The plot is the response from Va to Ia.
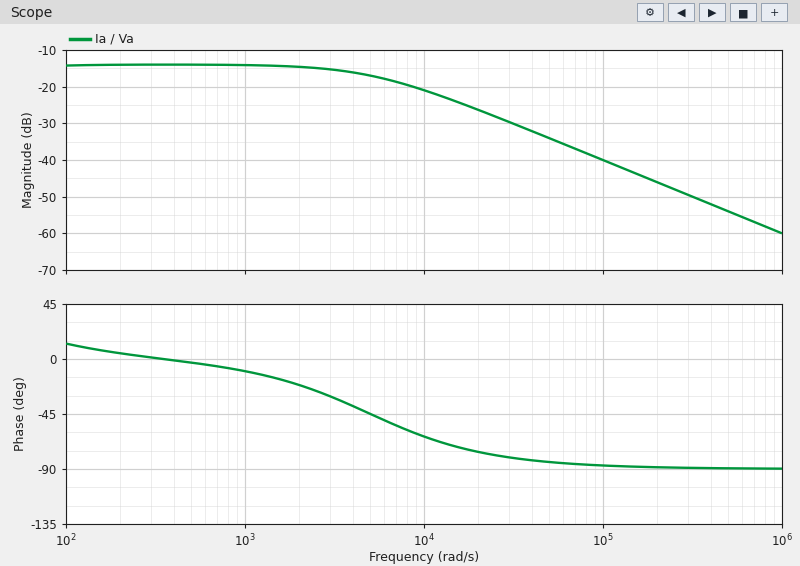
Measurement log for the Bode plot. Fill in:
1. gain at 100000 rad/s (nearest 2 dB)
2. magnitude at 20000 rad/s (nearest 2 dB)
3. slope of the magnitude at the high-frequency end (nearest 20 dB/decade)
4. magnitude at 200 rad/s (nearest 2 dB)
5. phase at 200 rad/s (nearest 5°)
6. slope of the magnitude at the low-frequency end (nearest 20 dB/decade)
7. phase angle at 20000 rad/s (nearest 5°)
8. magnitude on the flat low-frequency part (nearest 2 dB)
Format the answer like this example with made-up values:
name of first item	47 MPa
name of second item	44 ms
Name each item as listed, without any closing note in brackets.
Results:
gain at 100000 rad/s	-40 dB
magnitude at 20000 rad/s	-26 dB
slope of the magnitude at the high-frequency end	-20 dB/decade
magnitude at 200 rad/s	-14 dB
phase at 200 rad/s	5°
slope of the magnitude at the low-frequency end	0 dB/decade
phase angle at 20000 rad/s	-75°
magnitude on the flat low-frequency part	-14 dB
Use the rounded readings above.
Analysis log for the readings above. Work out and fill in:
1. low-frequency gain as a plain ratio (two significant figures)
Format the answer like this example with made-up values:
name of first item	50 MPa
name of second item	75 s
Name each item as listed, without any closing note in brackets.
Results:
low-frequency gain as a plain ratio	0.20
